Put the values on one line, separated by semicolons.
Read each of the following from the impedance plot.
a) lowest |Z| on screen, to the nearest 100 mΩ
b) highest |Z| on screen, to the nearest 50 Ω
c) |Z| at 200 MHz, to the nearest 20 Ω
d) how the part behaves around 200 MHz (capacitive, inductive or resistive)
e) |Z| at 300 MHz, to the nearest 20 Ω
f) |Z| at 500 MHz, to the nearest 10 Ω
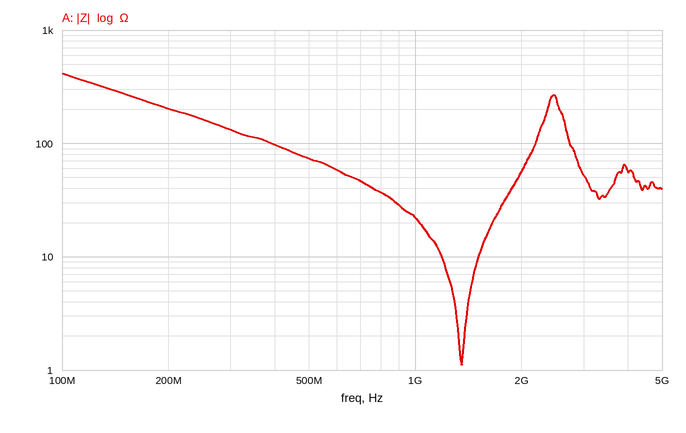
1.1 Ω; 400 Ω; 200 Ω; capacitive; 140 Ω; 70 Ω
